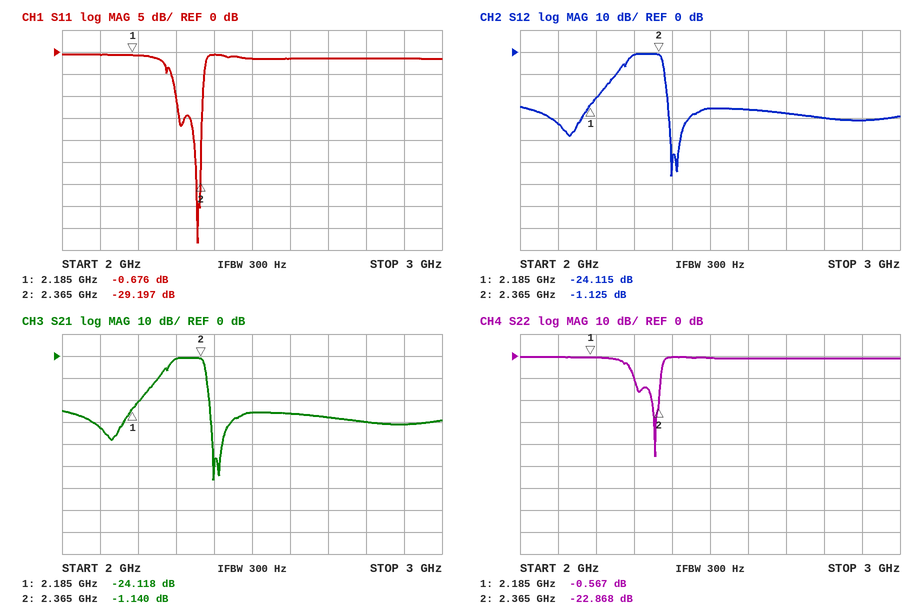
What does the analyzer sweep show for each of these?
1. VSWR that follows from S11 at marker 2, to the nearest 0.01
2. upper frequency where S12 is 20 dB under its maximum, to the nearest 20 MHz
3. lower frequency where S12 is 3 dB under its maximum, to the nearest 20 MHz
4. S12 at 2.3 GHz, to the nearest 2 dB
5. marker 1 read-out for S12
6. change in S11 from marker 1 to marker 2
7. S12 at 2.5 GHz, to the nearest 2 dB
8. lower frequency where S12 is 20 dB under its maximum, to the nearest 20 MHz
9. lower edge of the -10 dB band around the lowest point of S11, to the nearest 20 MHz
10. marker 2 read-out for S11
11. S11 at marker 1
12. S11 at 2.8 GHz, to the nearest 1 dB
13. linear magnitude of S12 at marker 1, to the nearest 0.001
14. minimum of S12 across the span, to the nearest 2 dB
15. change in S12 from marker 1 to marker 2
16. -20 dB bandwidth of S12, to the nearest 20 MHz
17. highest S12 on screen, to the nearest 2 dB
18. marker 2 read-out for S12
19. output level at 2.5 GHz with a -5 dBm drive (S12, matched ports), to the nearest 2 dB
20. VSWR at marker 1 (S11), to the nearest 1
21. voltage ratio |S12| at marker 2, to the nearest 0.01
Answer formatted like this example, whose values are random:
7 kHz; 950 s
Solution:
1.07; 2.38 GHz; 2.28 GHz; -2 dB; -24.115 dB; -28.521 dB; -26 dB; 2.20 GHz; 2.30 GHz; -29.197 dB; -0.676 dB; -1 dB; 0.062; -56 dB; 22.990 dB; 180 MHz; 0 dB; -1.125 dB; -30 dBm; 26; 0.88
